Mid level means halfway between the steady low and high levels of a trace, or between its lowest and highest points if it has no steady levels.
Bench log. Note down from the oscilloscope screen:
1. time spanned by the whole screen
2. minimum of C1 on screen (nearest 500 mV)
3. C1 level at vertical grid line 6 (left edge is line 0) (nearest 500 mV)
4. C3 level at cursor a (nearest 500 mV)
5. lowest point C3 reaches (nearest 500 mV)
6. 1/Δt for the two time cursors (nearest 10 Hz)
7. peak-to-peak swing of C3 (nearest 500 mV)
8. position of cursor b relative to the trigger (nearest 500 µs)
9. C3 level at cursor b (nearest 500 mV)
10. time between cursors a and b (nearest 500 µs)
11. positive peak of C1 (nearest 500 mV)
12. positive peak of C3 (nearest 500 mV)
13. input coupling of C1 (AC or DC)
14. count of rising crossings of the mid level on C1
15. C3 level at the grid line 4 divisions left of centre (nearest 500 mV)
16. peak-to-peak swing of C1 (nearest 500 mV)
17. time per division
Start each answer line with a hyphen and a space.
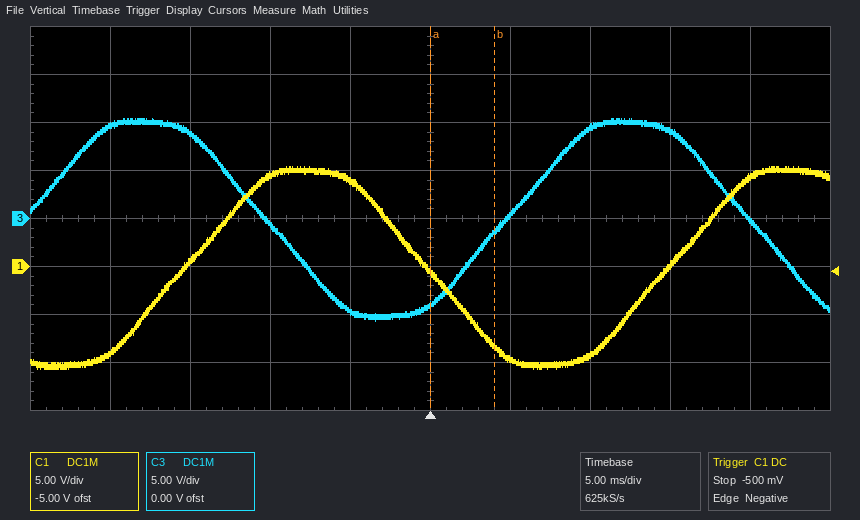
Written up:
- 50 ms
- -10.5 V
- -9.5 V
- -9.0 V
- -10.5 V
- 250 Hz
- 21.0 V
- +4.0 ms
- -1.5 V
- 4.0 ms
- 10.5 V
- 10.5 V
- DC
- 2
- 9.5 V
- 21.0 V
- 5 ms
